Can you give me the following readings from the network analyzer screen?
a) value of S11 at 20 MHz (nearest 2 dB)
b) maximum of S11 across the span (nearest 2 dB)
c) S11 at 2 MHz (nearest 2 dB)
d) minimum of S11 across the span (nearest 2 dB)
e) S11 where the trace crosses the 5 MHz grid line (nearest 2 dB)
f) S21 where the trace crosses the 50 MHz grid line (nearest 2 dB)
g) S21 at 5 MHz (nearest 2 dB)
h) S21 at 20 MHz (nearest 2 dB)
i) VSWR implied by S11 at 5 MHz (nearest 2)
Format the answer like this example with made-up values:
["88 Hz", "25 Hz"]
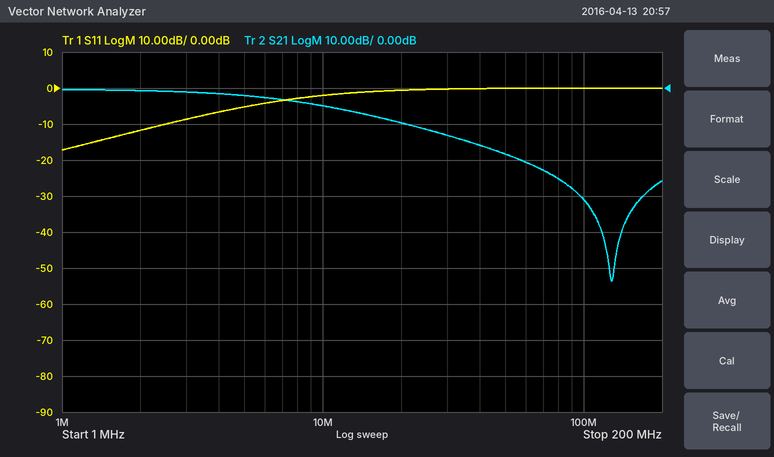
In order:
["0 dB", "0 dB", "-12 dB", "-18 dB", "-6 dB", "-18 dB", "-2 dB", "-10 dB", "4"]
